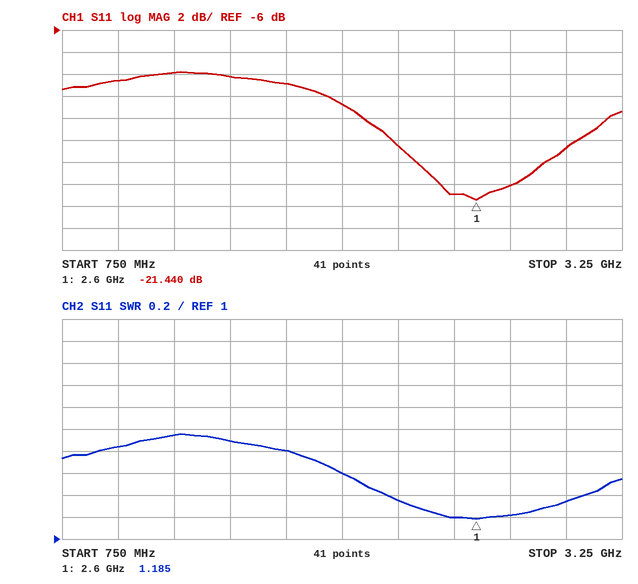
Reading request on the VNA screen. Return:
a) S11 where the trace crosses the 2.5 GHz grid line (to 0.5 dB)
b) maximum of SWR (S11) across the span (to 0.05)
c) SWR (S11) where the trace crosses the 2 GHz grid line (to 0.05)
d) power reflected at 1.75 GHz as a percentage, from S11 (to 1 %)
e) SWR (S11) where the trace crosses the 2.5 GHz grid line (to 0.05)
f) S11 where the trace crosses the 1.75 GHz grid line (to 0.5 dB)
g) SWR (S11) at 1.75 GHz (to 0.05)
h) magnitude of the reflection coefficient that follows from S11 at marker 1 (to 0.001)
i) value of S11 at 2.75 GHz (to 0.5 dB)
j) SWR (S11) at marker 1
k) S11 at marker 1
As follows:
-21.0 dB
1.95
1.60
8 %
1.20
-11.0 dB
1.80
0.085
-20.0 dB
1.185
-21.440 dB
